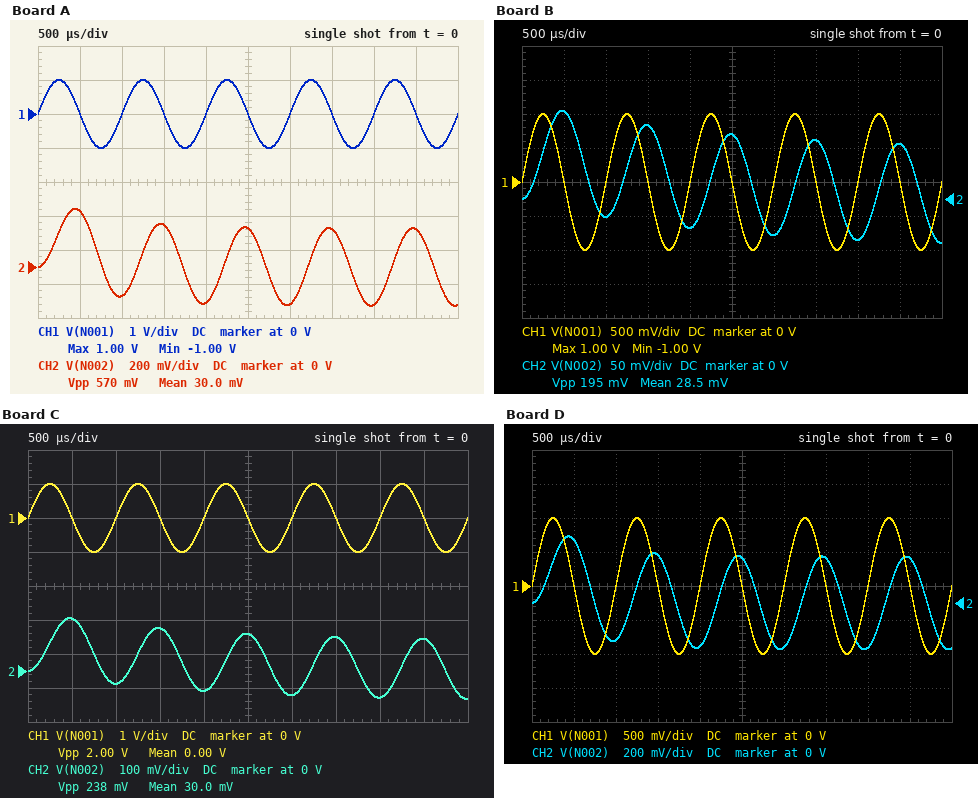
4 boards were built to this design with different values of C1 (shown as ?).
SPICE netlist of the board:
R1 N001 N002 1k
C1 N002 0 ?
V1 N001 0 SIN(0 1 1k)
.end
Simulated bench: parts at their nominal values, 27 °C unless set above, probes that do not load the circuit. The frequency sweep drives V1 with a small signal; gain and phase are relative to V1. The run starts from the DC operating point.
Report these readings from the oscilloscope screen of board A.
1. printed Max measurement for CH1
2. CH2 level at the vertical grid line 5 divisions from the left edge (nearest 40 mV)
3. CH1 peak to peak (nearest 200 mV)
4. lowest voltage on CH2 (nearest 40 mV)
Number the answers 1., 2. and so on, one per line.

1. 1.00 V
2. 240 mV
3. 2.0 V
4. -240 mV
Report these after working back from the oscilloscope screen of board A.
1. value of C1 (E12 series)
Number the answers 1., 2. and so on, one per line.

1. 680 nF
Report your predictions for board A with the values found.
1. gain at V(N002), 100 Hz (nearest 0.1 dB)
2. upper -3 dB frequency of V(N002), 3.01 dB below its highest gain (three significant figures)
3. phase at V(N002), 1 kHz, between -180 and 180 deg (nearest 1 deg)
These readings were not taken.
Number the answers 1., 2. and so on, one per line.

1. -0.7 dB
2. 234 Hz
3. -77 deg
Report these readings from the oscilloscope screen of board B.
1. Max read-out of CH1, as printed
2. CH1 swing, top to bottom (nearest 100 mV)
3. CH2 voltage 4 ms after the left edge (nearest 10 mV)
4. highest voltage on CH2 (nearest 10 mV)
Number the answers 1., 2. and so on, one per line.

1. 1.00 V
2. 2.0 V
3. -60 mV
4. 130 mV
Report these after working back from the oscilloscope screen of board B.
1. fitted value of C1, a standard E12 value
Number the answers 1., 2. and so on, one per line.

1. 2.2 µF
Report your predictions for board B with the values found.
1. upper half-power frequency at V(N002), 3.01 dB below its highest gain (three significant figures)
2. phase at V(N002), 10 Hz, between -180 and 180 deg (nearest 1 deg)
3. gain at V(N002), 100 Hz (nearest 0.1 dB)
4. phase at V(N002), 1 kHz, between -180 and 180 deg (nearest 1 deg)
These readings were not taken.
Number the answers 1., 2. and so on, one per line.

1. 72.3 Hz
2. -8 deg
3. -4.6 dB
4. -86 deg
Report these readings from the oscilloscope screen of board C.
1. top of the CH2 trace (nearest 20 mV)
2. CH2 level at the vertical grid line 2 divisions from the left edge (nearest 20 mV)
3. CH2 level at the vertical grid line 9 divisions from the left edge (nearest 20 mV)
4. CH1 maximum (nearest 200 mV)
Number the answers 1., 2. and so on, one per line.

1. 160 mV
2. -40 mV
3. 100 mV
4. 1.0 V
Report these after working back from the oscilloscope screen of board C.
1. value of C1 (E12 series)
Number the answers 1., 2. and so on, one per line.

1. 1.8 µF
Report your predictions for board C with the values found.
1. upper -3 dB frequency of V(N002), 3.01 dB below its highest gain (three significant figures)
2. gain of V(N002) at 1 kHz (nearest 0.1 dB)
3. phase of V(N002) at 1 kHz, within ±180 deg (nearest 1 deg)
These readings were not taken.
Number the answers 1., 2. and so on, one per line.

1. 88.4 Hz
2. -21.1 dB
3. -85 deg
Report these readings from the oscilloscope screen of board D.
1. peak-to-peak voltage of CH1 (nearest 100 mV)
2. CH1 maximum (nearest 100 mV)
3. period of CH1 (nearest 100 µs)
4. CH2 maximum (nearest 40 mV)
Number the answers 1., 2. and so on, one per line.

1. 2.0 V
2. 1.0 V
3. 1.0 ms
4. 400 mV
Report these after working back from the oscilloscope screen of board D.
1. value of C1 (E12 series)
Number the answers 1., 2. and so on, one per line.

1. 560 nF
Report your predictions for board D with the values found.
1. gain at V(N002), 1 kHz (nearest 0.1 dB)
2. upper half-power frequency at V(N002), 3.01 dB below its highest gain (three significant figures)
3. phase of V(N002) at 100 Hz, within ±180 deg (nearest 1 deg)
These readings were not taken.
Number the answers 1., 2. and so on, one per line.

1. -11.3 dB
2. 284 Hz
3. -19 deg
